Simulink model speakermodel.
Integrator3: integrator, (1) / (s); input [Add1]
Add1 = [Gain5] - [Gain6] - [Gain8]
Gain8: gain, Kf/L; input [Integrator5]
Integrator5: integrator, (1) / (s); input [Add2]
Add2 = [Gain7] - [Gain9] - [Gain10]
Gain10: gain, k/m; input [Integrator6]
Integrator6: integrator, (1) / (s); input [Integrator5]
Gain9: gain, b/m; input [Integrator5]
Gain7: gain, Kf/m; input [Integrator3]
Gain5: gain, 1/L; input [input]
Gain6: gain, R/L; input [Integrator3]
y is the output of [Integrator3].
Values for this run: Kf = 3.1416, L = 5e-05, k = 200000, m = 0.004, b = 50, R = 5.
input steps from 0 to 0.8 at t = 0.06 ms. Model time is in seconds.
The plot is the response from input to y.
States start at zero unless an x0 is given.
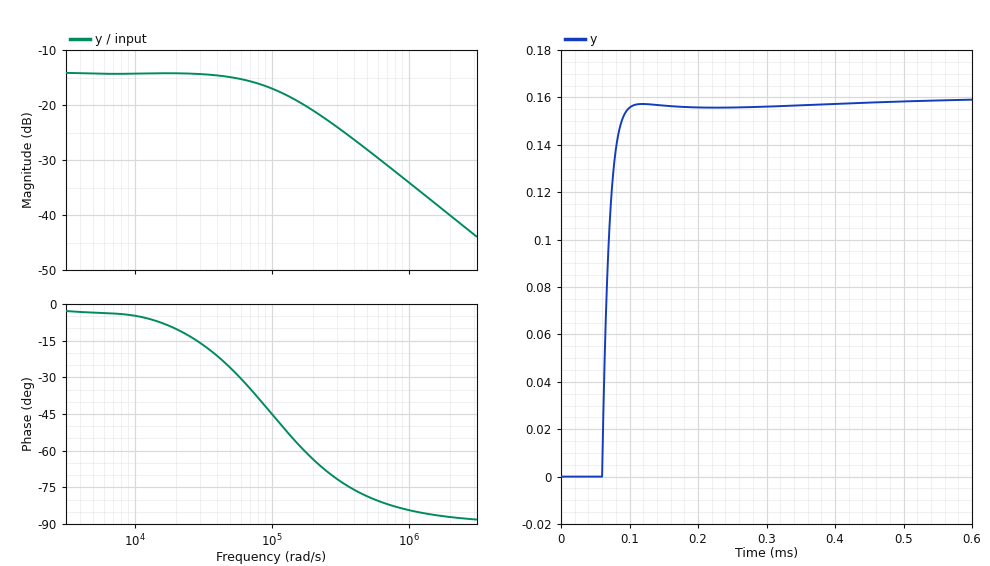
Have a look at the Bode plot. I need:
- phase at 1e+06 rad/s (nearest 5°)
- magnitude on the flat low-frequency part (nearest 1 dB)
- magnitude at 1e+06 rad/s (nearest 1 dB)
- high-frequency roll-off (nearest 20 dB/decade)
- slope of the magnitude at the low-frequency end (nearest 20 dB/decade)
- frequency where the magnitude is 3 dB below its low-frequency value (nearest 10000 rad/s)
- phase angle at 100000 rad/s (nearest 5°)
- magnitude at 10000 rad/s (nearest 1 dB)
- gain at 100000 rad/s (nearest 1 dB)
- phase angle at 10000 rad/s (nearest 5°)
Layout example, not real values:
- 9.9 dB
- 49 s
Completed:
- -85°
- -14 dB
- -34 dB
- -20 dB/decade
- 0 dB/decade
- 110000 rad/s
- -45°
- -14 dB
- -17 dB
- -5°
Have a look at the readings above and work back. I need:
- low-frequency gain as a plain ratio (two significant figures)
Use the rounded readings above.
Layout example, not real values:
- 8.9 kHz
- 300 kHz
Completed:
- 0.20
